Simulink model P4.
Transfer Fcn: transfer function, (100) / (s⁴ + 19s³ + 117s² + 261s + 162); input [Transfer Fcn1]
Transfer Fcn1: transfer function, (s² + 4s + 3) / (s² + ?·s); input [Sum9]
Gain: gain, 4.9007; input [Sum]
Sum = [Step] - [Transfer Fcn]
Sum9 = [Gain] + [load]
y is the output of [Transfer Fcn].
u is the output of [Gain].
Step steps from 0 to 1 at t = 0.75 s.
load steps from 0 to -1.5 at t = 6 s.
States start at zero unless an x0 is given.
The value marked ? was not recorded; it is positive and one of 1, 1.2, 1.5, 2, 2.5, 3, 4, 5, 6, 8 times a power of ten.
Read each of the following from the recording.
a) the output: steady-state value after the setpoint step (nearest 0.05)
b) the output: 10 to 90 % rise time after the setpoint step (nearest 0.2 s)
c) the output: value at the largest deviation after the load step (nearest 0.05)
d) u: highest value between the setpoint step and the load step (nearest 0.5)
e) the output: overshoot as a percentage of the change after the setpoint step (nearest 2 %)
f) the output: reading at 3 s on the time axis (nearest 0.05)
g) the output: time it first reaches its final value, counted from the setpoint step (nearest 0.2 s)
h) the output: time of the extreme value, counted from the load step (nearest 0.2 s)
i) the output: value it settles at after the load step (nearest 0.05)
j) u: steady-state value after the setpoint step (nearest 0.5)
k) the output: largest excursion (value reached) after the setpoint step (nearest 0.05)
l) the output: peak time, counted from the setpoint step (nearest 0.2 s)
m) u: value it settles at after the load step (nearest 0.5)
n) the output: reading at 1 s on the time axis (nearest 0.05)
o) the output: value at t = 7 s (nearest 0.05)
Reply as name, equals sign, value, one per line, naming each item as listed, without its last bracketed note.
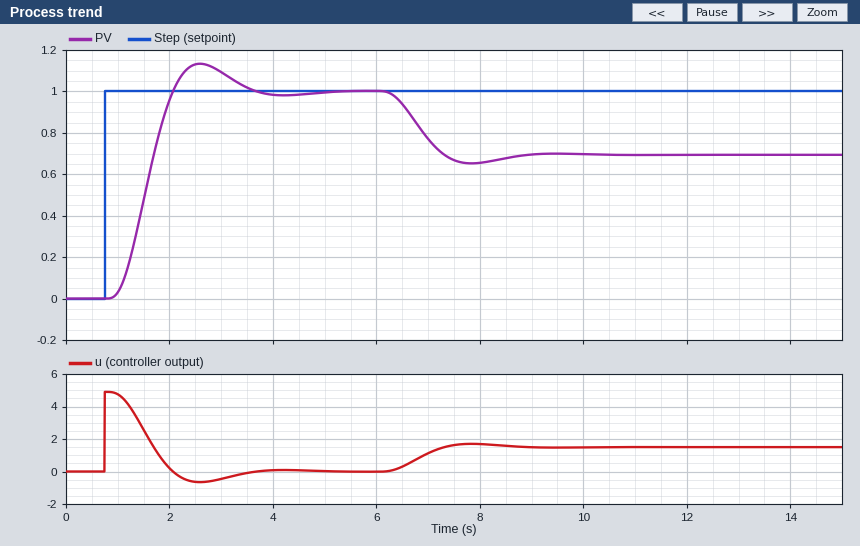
the output: steady-state value after the setpoint step = 1.00
the output: 10 to 90 % rise time after the setpoint step = 0.8 s
the output: value at the largest deviation after the load step = 0.65
u: highest value between the setpoint step and the load step = 5.0
the output: overshoot as a percentage of the change after the setpoint step = 14 %
the output: reading at 3 s on the time axis = 1.10
the output: time it first reaches its final value, counted from the setpoint step = 1.4 s
the output: time of the extreme value, counted from the load step = 1.8 s
the output: value it settles at after the load step = 0.70
u: steady-state value after the setpoint step = 0.0
the output: largest excursion (value reached) after the setpoint step = 1.15
the output: peak time, counted from the setpoint step = 1.8 s
u: value it settles at after the load step = 1.5
the output: reading at 1 s on the time axis = 0.05
the output: value at t = 7 s = 0.75
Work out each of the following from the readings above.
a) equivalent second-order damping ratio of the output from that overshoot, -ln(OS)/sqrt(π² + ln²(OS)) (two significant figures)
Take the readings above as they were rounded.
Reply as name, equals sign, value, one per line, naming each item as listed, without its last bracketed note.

equivalent second-order damping ratio of the output from that overshoot, -ln(OS)/sqrt(π² + ln²(OS)) = 0.53
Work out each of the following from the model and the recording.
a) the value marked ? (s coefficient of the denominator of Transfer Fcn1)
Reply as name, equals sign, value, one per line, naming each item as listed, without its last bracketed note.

the value marked ? = 6
